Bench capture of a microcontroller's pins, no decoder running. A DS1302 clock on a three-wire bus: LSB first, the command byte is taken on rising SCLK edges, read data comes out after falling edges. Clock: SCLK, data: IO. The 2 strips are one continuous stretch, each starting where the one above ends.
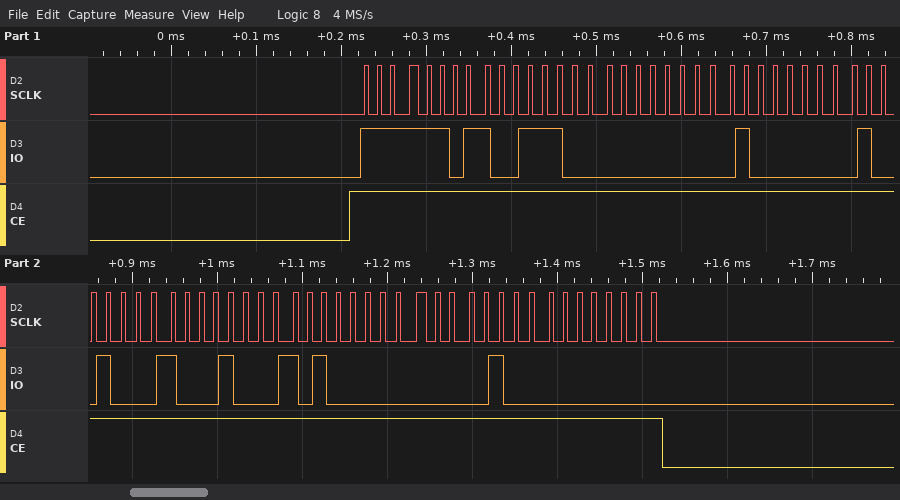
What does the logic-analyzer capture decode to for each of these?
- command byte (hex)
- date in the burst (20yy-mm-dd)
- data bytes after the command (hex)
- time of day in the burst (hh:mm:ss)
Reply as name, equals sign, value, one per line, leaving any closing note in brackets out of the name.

command byte = 0xBF
date in the burst = 2020-11-12
data bytes after the command = 39 00 02 12 11 05 20 00
time of day in the burst = 02:00:39
